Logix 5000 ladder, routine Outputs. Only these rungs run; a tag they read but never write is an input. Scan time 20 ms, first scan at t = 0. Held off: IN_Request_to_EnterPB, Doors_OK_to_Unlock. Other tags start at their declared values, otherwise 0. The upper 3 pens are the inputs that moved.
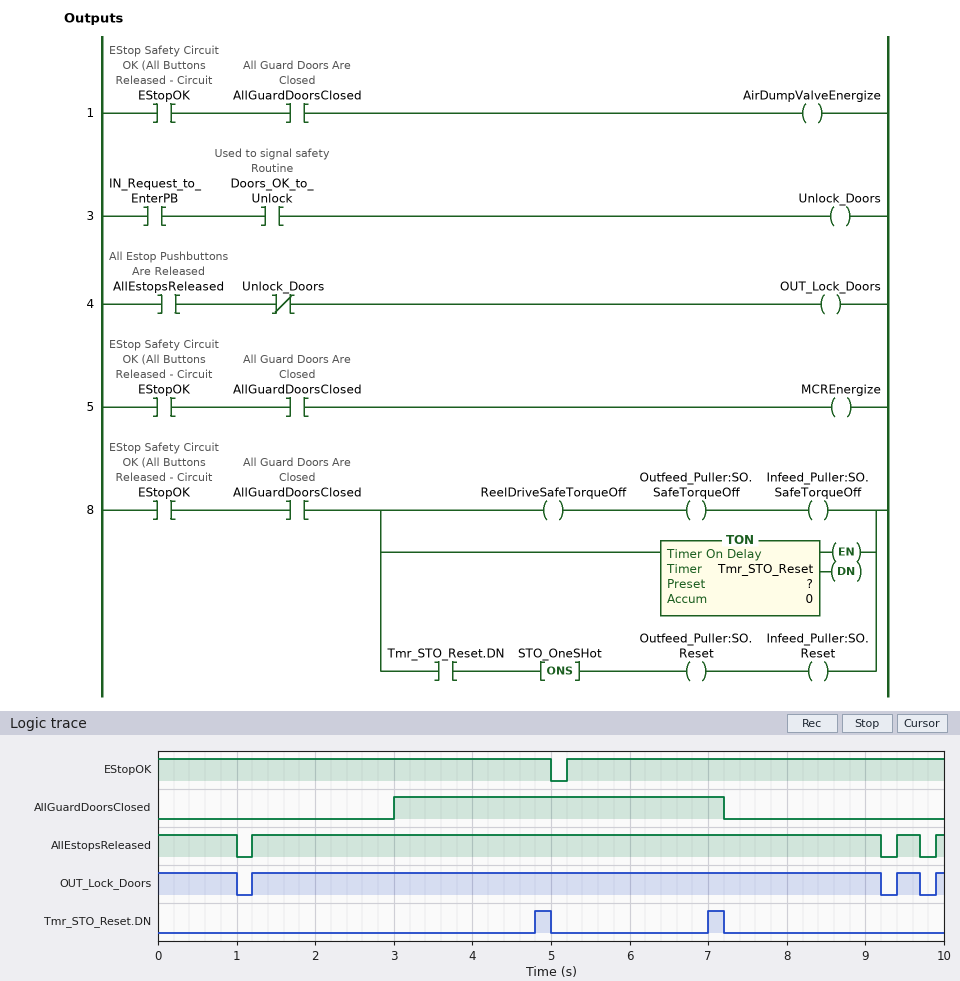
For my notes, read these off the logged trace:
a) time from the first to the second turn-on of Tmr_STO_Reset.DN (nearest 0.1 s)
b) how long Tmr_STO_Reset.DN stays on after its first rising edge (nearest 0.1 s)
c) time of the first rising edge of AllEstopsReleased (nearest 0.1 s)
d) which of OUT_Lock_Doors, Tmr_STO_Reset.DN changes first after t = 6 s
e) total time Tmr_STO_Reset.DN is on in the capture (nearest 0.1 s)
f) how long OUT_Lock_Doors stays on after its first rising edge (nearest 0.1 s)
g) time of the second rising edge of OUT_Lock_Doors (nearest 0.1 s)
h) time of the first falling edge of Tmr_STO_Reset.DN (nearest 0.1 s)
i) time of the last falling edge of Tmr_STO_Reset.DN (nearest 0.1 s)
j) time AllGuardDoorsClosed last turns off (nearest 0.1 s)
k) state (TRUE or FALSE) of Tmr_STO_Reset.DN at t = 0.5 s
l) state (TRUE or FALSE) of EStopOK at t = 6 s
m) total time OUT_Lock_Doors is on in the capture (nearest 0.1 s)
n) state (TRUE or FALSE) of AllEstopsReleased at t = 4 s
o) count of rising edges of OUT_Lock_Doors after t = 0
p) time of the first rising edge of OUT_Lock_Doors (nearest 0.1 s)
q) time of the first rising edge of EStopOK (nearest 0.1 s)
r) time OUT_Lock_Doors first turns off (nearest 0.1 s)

2.2 s
0.2 s
1.2 s
Tmr_STO_Reset.DN
0.4 s
8.0 s
9.4 s
5.0 s
7.2 s
7.2 s
FALSE
TRUE
9.4 s
TRUE
3
1.2 s
5.2 s
1.0 s
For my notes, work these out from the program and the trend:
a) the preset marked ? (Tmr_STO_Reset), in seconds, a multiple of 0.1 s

1.8 s
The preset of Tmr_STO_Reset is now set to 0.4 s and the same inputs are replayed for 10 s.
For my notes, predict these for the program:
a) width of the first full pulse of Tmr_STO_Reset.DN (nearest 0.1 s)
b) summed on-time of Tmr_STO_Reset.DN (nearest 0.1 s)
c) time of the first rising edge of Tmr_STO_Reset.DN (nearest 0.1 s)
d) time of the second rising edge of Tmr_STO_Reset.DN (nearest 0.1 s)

1.6 s
3.2 s
3.4 s
5.6 s
